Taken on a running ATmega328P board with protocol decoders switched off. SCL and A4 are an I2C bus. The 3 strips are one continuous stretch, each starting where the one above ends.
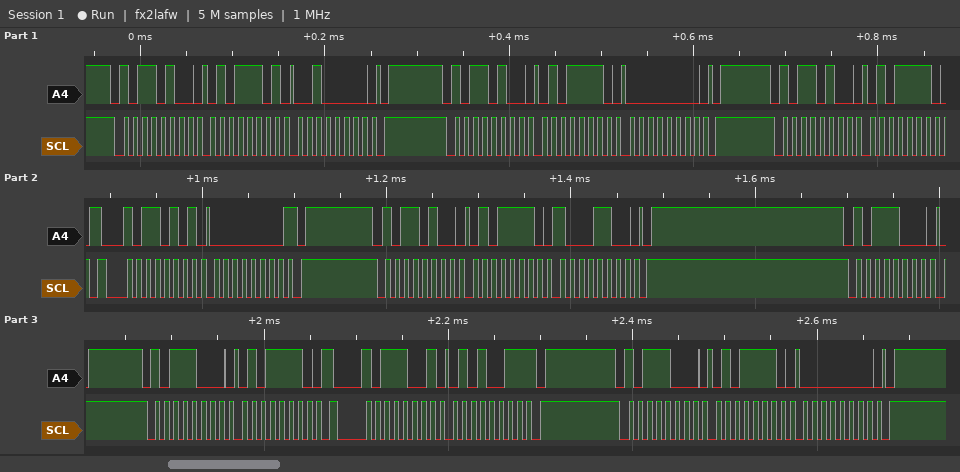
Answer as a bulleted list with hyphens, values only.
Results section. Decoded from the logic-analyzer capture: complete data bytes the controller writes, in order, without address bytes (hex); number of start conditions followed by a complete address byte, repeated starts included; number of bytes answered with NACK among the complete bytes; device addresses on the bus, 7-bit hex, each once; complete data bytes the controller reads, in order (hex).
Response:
- 5D 20 5E 00 5E 5E 8C 5E 5E 00
- 9
- 2
- 0x5A 0x5C
- 00 53
